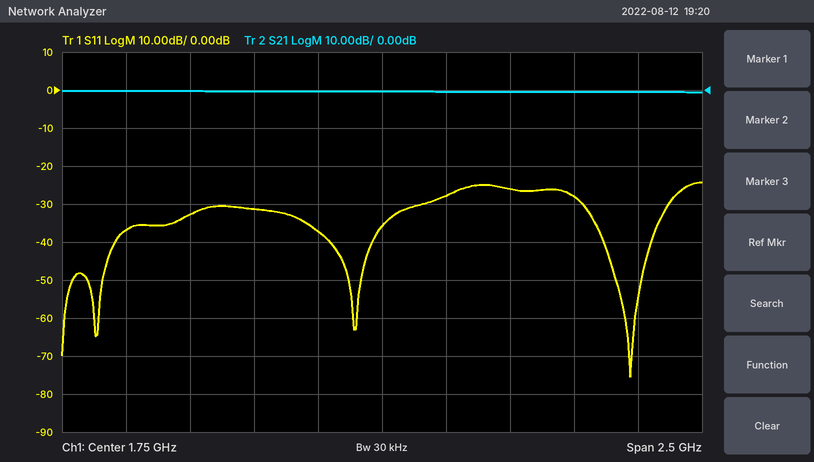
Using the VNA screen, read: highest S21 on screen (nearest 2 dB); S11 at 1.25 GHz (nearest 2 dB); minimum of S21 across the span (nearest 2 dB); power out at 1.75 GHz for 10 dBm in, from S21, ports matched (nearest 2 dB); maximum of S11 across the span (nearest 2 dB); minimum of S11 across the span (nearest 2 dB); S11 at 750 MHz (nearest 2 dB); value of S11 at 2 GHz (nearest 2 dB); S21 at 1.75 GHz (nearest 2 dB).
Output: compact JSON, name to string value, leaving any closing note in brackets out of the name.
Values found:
{"highest S21 on screen": "0 dB", "S11 at 1.25 GHz": "-32 dB", "minimum of S21 across the span": "0 dB", "power out at 1.75 GHz for 10 dBm in, from S21, ports matched": "10 dBm", "maximum of S11 across the span": "-24 dB", "minimum of S11 across the span": "-76 dB", "S11 at 750 MHz": "-36 dB", "value of S11 at 2 GHz": "-28 dB", "S21 at 1.75 GHz": "0 dB"}
